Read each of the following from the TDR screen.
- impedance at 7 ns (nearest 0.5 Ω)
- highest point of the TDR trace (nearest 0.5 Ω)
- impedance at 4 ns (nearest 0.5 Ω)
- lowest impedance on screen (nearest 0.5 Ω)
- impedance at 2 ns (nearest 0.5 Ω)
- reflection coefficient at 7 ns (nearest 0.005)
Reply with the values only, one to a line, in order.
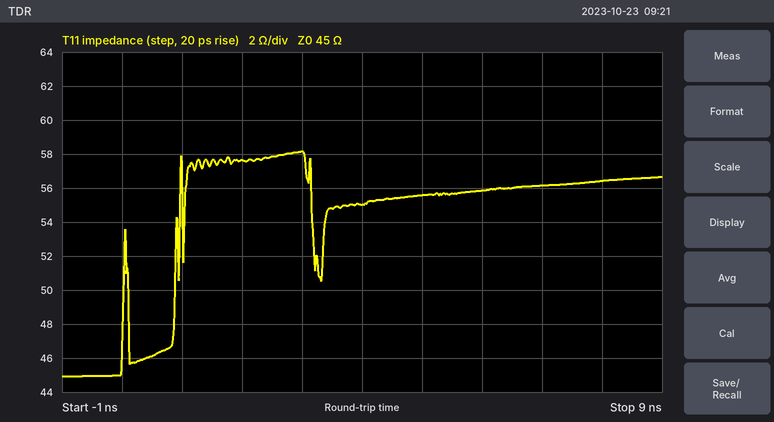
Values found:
56.0 Ω
58.0 Ω
55.0 Ω
45.0 Ω
57.5 Ω
+0.110
